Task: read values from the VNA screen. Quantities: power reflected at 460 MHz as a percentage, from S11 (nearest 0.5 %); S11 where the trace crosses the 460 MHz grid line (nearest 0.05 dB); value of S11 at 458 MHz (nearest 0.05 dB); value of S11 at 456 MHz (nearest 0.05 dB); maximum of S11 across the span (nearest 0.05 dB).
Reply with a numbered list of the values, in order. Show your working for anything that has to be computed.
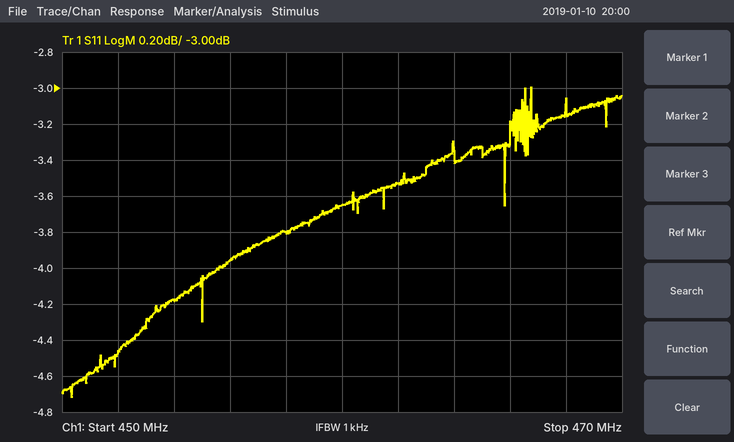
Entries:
1. 10^(-3.65/10) ≈ 43.2 %, so 43.0 % to the nearest 0.5 %
2. -3.65 dB
3. -3.80 dB
4. -3.95 dB
5. -3.00 dB
